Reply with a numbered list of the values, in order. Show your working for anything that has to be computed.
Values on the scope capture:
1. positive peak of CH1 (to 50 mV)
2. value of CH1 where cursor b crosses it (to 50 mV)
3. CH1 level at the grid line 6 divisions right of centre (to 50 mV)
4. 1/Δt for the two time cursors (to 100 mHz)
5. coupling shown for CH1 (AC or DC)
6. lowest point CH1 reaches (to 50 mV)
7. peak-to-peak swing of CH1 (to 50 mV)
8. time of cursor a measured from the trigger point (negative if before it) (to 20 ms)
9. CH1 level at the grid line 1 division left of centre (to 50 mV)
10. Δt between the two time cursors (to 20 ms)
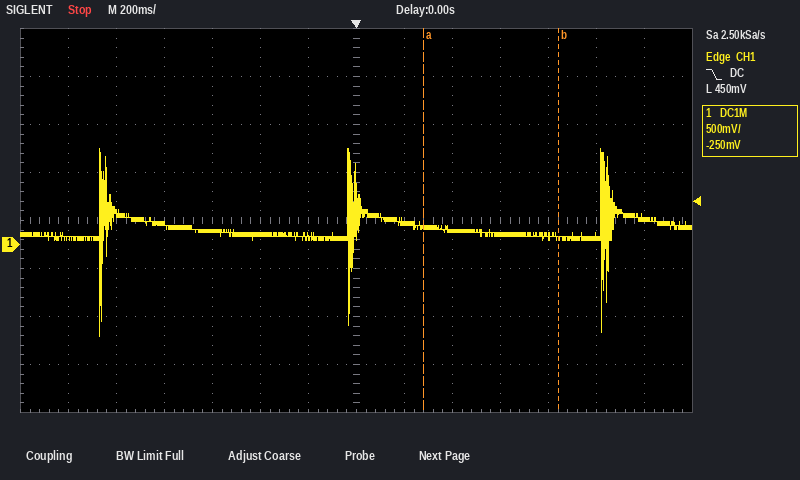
1. 1.00 V
2. 100 mV
3. 250 mV
4. 1 / 560 ms ≈ 1.8 Hz
5. DC
6. -950 mV
7. 1.00 V − (-950 mV) = 1.95 V
8. +280 ms
9. 100 mV
10. 560 ms
